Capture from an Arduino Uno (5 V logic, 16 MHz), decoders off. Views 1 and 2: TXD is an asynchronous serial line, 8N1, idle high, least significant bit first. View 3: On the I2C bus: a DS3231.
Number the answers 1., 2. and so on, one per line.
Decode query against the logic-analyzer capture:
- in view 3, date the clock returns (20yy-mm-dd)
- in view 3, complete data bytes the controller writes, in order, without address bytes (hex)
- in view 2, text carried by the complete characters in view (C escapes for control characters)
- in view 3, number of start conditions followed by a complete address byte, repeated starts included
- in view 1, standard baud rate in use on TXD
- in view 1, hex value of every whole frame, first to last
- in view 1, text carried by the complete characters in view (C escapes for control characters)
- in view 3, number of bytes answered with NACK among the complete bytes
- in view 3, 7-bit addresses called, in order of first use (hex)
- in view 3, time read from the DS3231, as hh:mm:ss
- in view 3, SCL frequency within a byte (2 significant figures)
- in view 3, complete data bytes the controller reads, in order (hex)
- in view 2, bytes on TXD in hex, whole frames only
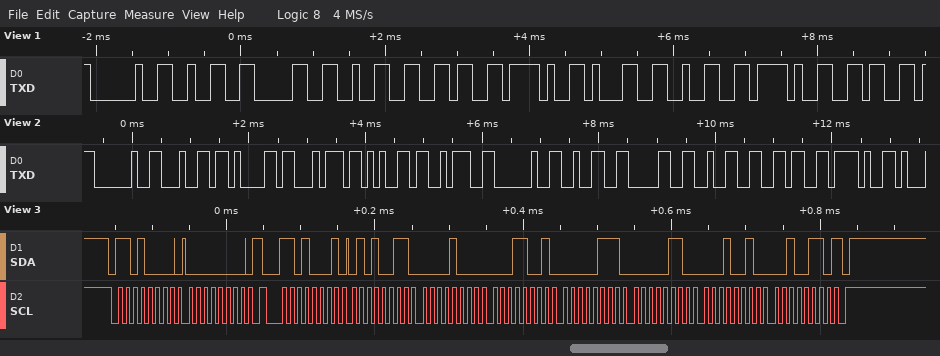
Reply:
1. 2026-12-06
2. 00
3. " date: 2026/"
4. 2
5. 9600 baud
6. 20 32 30 32 36 2F 31 32 2F 36
7. " 2026/12/6"
8. 1
9. 0x68
10. 19:08:53
11. 100 kHz
12. 53 08 19 07 06 12 26
13. 20 64 61 74 65 3A 20 32 30 32 36 2F
